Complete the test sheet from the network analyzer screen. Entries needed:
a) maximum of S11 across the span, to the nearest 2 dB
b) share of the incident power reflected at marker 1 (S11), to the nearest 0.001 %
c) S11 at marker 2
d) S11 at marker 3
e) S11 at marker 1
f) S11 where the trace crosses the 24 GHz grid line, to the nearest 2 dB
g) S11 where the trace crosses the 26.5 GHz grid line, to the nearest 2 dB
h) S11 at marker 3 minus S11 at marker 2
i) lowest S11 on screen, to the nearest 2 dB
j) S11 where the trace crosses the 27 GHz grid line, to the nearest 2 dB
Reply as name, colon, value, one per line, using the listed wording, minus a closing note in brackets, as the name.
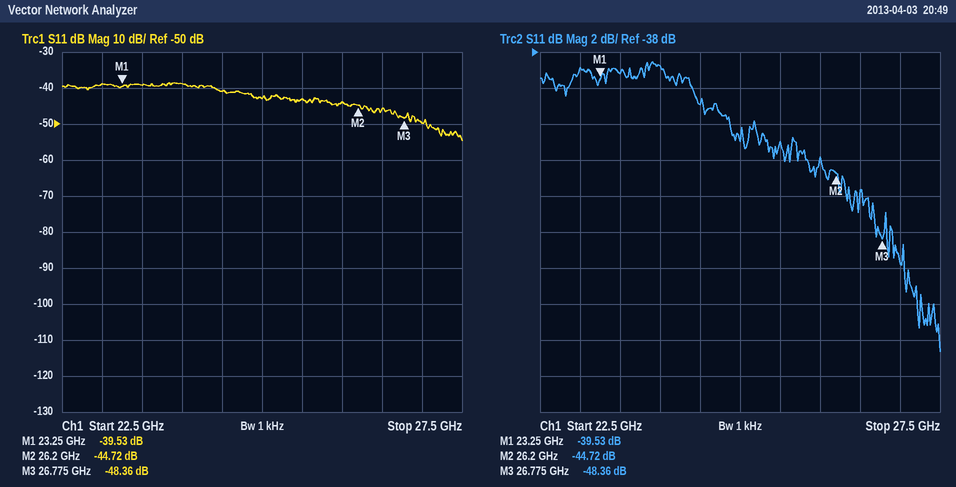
maximum of S11 across the span, to the nearest 2 dB: -38 dB
share of the incident power reflected at marker 1 (S11), to the nearest 0.001 %: 0.011 %
S11 at marker 2: -44.72 dB
S11 at marker 3: -48.36 dB
S11 at marker 1: -39.53 dB
S11 where the trace crosses the 24 GHz grid line, to the nearest 2 dB: -38 dB
S11 where the trace crosses the 26.5 GHz grid line, to the nearest 2 dB: -46 dB
S11 at marker 3 minus S11 at marker 2: -3.64 dB
lowest S11 on screen, to the nearest 2 dB: -54 dB
S11 where the trace crosses the 27 GHz grid line, to the nearest 2 dB: -50 dB
